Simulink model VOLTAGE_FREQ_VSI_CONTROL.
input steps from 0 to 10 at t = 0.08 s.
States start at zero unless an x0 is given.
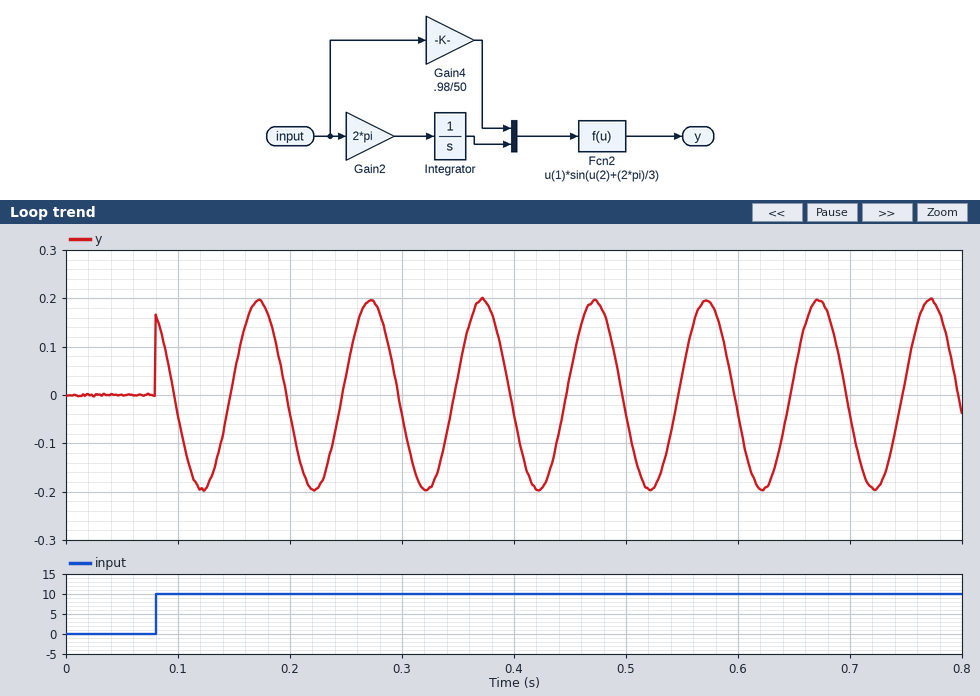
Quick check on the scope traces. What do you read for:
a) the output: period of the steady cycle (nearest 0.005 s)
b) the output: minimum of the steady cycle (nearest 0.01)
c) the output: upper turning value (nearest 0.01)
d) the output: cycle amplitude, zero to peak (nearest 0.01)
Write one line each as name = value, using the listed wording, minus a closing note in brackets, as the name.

the output: period of the steady cycle = 0.100 s
the output: minimum of the steady cycle = -0.20
the output: upper turning value = 0.20
the output: cycle amplitude, zero to peak = 0.20
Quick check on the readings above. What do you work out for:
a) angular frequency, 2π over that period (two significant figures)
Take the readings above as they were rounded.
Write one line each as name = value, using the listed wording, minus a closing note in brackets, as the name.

angular frequency, 2π over that period = 63 rad/s
